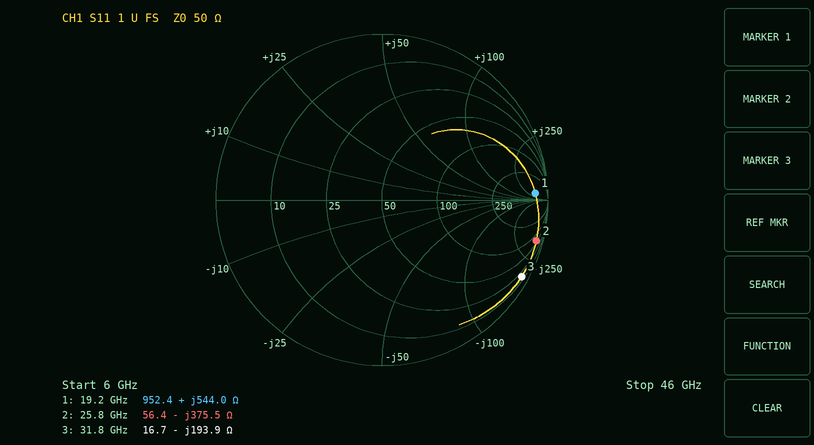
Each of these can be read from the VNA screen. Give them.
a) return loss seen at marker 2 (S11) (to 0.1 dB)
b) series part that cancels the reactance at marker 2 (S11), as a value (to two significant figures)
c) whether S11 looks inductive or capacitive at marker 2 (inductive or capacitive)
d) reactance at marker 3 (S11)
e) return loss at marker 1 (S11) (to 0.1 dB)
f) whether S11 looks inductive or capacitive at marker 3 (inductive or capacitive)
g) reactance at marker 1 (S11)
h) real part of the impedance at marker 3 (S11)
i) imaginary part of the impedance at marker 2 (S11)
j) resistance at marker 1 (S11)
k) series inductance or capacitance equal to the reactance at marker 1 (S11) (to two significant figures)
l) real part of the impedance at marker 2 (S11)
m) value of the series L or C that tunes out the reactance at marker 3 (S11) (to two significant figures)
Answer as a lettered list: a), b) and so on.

a) 0.3 dB
b) 2.3 nH
c) capacitive
d) -193.9 Ω
e) 0.7 dB
f) capacitive
g) +544.0 Ω
h) 16.7 Ω
i) -375.5 Ω
j) 952.4 Ω
k) 4.5 nH
l) 56.4 Ω
m) 970 pH
